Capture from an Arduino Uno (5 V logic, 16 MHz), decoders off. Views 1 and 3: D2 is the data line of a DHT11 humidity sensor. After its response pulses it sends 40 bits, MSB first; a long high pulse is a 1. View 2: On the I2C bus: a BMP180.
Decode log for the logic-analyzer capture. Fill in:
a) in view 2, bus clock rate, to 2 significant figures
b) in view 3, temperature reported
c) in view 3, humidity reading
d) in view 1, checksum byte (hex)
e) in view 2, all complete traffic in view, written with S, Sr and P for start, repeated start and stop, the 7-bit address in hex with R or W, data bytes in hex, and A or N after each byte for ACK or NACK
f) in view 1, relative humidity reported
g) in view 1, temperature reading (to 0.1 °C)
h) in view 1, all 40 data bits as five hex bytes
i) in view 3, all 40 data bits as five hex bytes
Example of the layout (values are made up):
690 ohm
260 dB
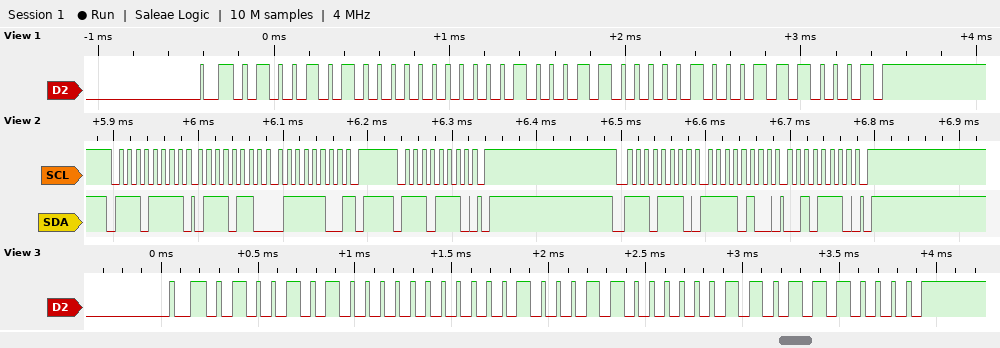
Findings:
100 kHz
35.3 °C
74 %
0x71
S 77R A 76 A 7C N P S 77W A P S 77W A F4 A 2E A P
74 %
35.4 °C
4A 00 23 04 71
4A 00 23 03 70
